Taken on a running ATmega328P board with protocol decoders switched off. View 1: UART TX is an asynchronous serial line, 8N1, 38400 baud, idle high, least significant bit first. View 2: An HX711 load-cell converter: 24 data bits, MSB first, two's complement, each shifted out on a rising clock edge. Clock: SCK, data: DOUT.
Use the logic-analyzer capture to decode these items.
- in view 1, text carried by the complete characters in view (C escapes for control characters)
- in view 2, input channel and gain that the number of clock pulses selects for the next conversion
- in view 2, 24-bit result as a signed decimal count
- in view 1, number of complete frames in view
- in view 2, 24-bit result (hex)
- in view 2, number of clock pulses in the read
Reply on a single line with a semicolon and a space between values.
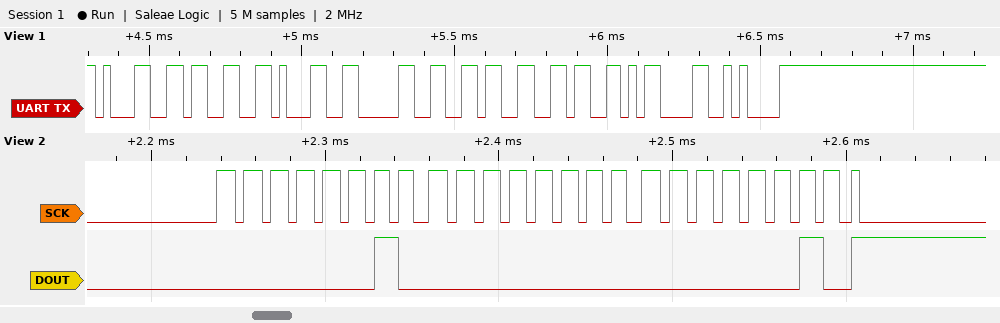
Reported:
"131066\r\n"; channel A, gain 128; 131074; 8; 0x020002; 25
